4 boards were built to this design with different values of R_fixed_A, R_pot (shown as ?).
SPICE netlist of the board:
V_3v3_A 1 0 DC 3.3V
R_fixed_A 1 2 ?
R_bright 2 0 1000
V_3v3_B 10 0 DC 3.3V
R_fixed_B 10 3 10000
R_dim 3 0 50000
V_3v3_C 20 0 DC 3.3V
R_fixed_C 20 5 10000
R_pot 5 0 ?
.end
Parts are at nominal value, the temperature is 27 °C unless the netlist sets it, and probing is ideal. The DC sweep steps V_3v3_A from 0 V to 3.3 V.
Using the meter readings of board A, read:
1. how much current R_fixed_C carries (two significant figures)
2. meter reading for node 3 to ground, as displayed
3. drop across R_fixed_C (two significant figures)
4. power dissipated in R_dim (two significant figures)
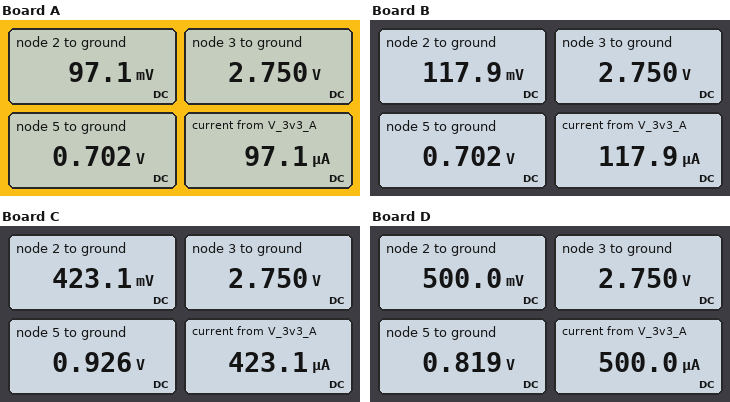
260 µA
2.750 V
2.6 V
150 µW
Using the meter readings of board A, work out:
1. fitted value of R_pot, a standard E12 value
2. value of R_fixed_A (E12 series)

2.7 kΩ
33 kΩ
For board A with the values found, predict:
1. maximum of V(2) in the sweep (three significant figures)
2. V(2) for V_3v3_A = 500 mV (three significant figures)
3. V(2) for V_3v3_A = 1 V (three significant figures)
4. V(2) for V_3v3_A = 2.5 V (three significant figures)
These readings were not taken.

97.1 mV
14.7 mV
29.4 mV
73.5 mV
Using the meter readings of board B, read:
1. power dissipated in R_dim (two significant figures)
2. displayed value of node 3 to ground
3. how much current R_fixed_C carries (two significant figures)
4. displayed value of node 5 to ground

150 µW
2.750 V
260 µA
0.702 V
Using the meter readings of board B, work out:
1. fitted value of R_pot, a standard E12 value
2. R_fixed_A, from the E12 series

2.7 kΩ
27 kΩ
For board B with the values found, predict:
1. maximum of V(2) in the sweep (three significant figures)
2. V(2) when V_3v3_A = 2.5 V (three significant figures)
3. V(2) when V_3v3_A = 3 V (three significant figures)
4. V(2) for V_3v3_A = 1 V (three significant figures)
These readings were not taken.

118 mV
89.3 mV
107 mV
35.7 mV
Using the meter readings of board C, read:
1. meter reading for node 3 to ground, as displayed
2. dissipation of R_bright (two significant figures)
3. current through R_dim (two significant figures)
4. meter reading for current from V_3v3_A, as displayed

2.750 V
180 µW
55 µA
423.1 µA
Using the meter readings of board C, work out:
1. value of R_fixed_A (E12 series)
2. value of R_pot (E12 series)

6.8 kΩ
3.9 kΩ
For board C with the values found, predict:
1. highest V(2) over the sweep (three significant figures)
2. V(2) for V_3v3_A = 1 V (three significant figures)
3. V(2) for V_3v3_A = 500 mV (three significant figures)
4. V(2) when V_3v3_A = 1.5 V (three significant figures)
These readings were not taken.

423 mV
128 mV
64.1 mV
192 mV
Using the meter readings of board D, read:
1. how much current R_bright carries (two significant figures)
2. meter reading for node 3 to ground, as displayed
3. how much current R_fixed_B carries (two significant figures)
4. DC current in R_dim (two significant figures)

500 µA
2.750 V
55 µA
55 µA
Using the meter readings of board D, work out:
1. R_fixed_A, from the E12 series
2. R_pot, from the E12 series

5.6 kΩ
3.3 kΩ
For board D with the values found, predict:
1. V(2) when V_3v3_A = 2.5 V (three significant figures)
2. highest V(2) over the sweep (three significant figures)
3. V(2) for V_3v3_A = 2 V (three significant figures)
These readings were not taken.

379 mV
500 mV
303 mV
